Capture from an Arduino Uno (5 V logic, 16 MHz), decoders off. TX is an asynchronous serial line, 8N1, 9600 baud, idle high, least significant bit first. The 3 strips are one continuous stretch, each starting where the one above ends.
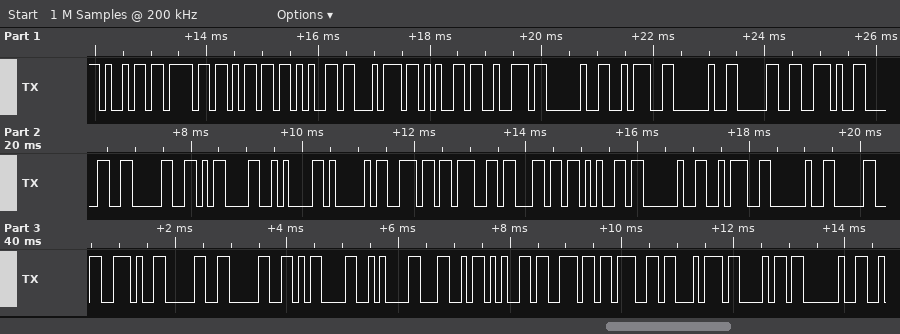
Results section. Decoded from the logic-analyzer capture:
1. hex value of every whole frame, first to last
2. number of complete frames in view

0x69 0x6F 0x6D 0x65 0x74 0x65 0x72 0x20 0x3A 0x20 0x30 0x2E 0x30 0x30 0x0D 0x0A 0x41 0x6E 0x67 0x6C 0x65 0x20 0x3A 0x20 0x30 0x2E 0x30 0x30 0x0D 0x0A 0x4C 0x65 0x6E 0x67 0x74 0x68 0x20
37
